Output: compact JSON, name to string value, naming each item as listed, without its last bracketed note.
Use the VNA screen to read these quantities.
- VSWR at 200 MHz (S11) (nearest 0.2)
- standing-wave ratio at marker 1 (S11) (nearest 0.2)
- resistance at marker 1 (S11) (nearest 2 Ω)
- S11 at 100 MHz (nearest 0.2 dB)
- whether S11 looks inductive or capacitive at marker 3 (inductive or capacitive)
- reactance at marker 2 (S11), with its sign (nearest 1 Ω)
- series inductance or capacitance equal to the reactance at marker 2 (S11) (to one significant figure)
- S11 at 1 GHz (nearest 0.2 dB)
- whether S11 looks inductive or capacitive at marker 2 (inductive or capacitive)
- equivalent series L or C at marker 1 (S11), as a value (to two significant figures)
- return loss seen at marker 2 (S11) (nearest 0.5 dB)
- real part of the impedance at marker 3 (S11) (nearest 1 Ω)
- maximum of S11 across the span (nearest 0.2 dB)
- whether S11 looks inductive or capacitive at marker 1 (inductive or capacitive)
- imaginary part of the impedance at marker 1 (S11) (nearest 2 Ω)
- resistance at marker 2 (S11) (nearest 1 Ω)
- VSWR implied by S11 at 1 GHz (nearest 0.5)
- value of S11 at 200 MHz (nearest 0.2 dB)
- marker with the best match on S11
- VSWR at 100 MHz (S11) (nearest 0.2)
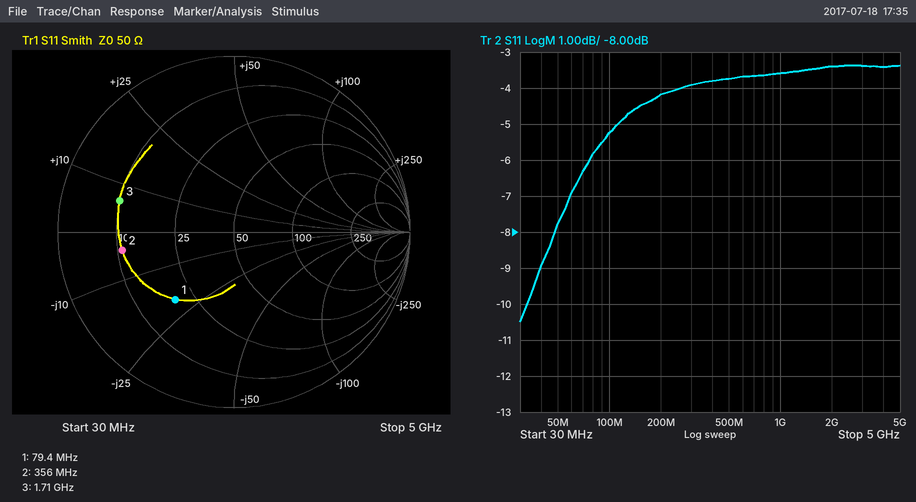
{"VSWR at 200 MHz (S11)": "4.2", "standing-wave ratio at marker 1 (S11)": "3.0", "resistance at marker 1 (S11)": "20 Ω", "S11 at 100 MHz": "-5.2 dB", "whether S11 looks inductive or capacitive at marker 3": "inductive", "reactance at marker 2 (S11), with its sign": "-4 Ω", "series inductance or capacitance equal to the reactance at marker 2 (S11)": "100 pF", "S11 at 1 GHz": "-3.6 dB", "whether S11 looks inductive or capacitive at marker 2": "capacitive", "equivalent series L or C at marker 1 (S11), as a value": "100 pF", "return loss seen at marker 2 (S11)": "4.0 dB", "real part of the impedance at marker 3 (S11)": "10 Ω", "maximum of S11 across the span": "-3.4 dB", "whether S11 looks inductive or capacitive at marker 1": "capacitive", "imaginary part of the impedance at marker 1 (S11)": "-20 Ω", "resistance at marker 2 (S11)": "11 Ω", "VSWR implied by S11 at 1 GHz": "5.0", "value of S11 at 200 MHz": "-4.2 dB", "marker with the best match on S11": "marker 1", "VSWR at 100 MHz (S11)": "3.4"}
